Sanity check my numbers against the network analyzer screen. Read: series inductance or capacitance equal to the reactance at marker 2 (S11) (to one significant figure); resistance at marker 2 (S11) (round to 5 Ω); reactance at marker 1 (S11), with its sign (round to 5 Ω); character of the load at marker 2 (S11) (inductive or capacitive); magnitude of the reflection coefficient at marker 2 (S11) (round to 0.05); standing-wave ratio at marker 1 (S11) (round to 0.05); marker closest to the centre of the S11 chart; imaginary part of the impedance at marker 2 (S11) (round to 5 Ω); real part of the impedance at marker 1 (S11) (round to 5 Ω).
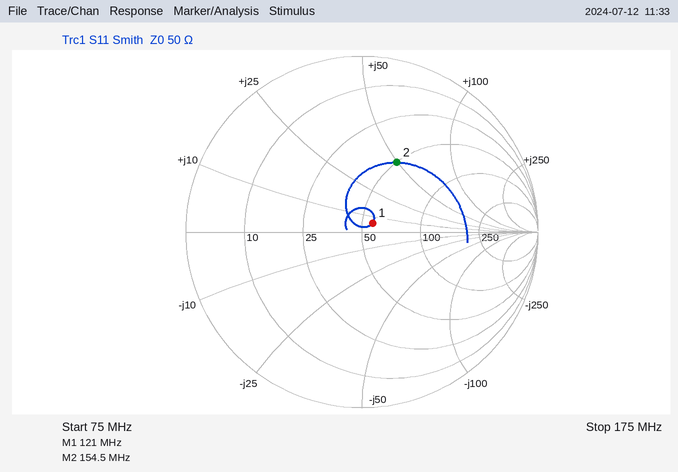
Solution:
50 nH
50 Ω
+5 Ω
inductive
0.45
1.15
marker 1
+50 Ω
55 Ω
